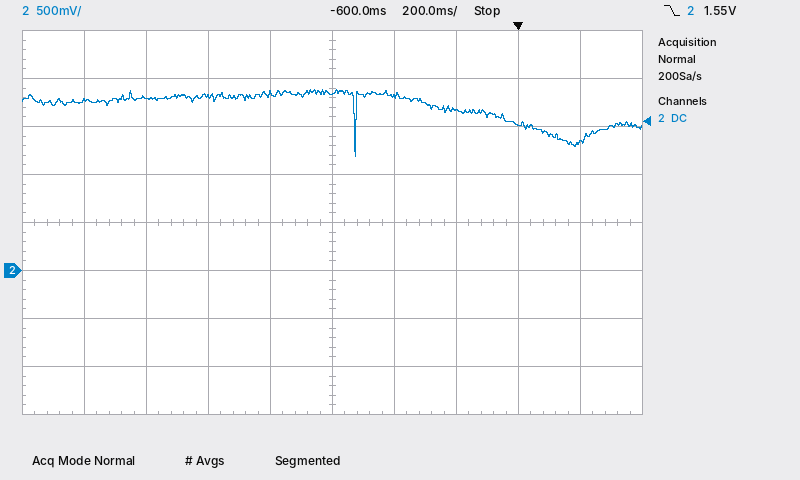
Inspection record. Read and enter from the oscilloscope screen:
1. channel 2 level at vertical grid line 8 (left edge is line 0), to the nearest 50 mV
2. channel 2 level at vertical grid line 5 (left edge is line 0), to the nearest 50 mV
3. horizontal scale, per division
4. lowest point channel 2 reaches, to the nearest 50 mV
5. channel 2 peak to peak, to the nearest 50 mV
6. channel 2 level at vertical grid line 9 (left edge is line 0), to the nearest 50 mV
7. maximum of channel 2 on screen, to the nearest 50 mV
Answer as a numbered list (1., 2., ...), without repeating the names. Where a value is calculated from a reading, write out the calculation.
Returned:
1. 1.50 V
2. 1.85 V
3. 200 ms
4. 1.20 V
5. 1.90 V − (1.20 V) = 700 mV
6. 1.35 V
7. 1.90 V
